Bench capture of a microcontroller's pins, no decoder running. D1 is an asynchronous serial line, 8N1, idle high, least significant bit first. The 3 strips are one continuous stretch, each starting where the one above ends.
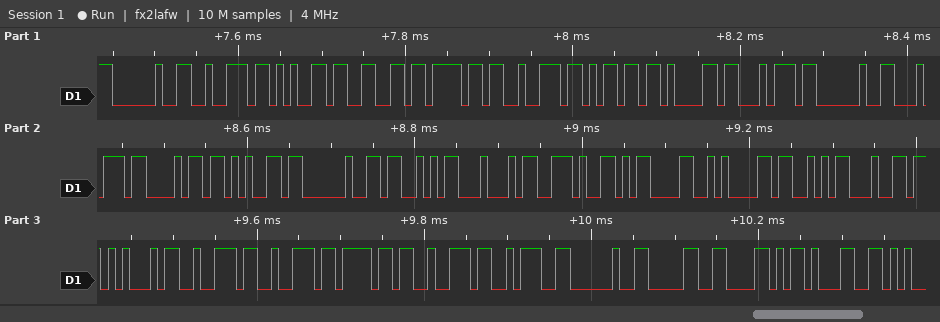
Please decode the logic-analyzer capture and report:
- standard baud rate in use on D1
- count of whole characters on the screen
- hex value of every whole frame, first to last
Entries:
115200 baud
31
20 72 65 66 6F 72 6D 61 74 20 74 68 65 20 53 44 2E 0D 0A 53 64 45 72 72 6F 72 3A 20 30 58 31
